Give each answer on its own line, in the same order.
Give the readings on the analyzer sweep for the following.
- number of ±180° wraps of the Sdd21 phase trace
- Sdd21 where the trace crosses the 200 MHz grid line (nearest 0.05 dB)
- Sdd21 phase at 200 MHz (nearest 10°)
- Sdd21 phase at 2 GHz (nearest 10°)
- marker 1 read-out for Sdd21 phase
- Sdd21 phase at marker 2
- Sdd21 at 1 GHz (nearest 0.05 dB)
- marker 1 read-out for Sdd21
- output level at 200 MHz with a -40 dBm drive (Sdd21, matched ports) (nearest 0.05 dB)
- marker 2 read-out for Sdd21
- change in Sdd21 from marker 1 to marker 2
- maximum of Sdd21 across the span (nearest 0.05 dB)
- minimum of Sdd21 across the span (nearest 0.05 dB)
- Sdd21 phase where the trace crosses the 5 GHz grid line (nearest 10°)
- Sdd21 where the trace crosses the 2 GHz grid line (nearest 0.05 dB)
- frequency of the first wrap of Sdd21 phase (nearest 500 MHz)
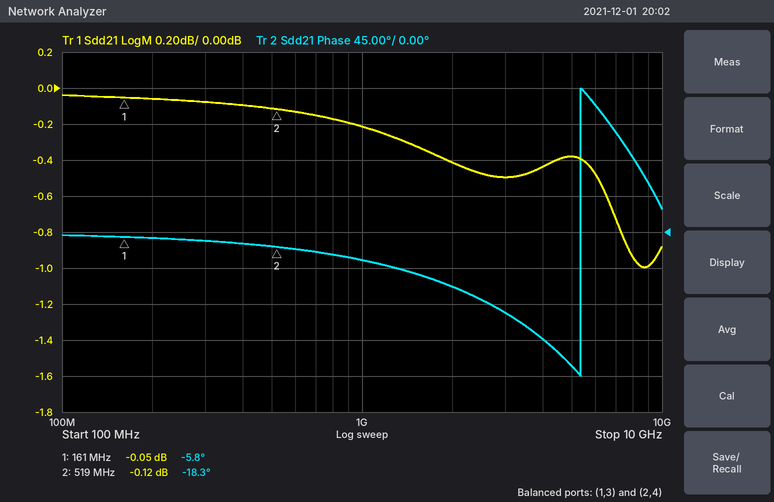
1
-0.05 dB
-10°
-70°
-5.8°
-18.3°
-0.20 dB
-0.05 dB
-40.05 dBm
-0.12 dB
-0.07 dB
-0.05 dB
-1.00 dB
-170°
-0.40 dB
5.5 GHz
